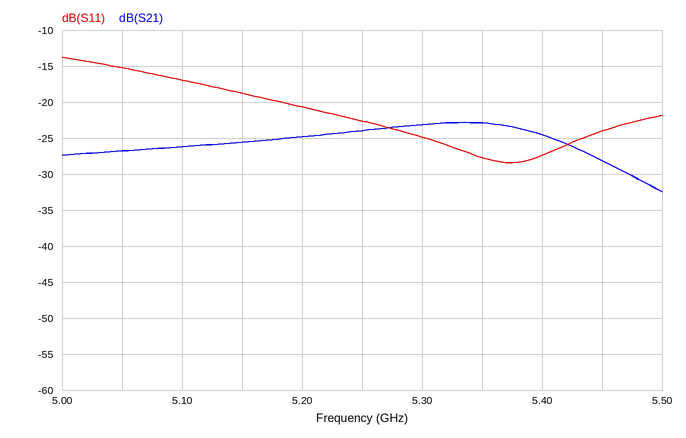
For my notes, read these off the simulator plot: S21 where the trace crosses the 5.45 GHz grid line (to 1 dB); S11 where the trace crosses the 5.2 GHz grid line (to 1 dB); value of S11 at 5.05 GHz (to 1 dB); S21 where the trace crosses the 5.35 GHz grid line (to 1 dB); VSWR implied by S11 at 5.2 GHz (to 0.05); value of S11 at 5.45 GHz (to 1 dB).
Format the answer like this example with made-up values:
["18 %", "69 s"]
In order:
["-28 dB", "-21 dB", "-15 dB", "-23 dB", "1.20", "-24 dB"]
